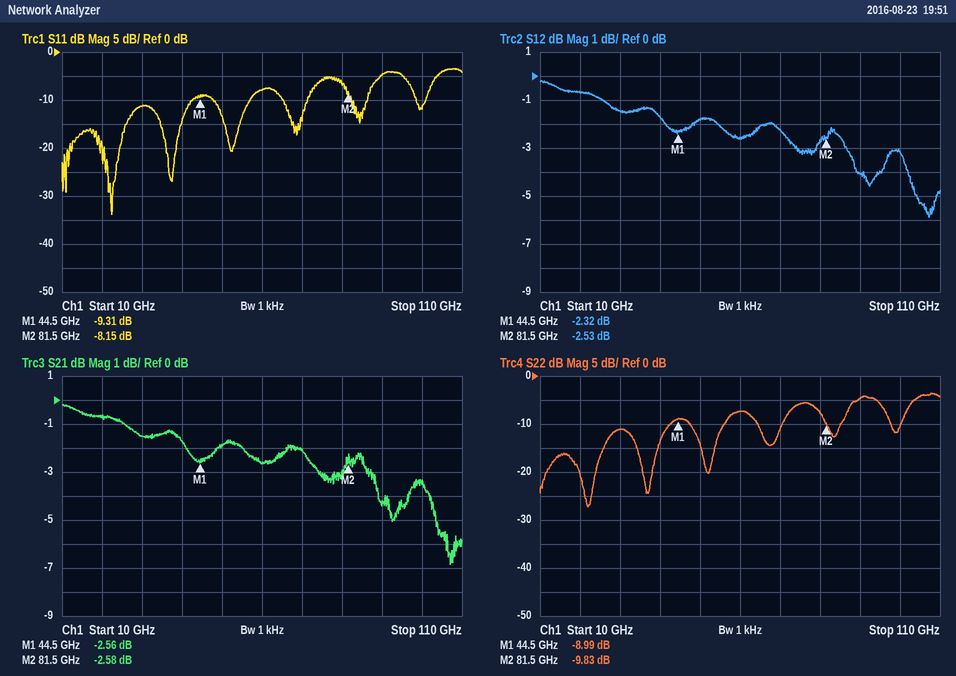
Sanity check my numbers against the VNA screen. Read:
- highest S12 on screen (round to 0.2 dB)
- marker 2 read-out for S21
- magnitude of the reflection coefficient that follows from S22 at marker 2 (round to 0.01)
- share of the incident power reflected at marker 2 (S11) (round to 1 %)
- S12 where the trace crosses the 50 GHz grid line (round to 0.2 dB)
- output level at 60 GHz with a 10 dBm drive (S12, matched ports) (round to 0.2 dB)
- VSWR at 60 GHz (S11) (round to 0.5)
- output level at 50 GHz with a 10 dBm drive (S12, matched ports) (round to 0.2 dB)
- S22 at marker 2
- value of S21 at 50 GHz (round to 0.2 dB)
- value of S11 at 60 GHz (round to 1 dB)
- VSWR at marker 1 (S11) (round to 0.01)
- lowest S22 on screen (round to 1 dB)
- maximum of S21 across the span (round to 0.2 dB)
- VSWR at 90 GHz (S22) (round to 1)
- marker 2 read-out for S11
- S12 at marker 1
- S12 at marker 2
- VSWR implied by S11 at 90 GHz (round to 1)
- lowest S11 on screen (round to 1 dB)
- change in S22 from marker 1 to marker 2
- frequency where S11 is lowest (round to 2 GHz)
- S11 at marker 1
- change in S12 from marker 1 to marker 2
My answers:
-0.2 dB
-2.58 dB
0.32
15 %
-1.8 dB
7.4 dBm
2.5
8.2 dBm
-9.83 dB
-1.8 dB
-8 dB
2.04
-27 dB
-0.2 dB
4
-8.15 dB
-2.32 dB
-2.53 dB
4
-34 dB
-0.84 dB
22 GHz
-9.31 dB
-0.21 dB
